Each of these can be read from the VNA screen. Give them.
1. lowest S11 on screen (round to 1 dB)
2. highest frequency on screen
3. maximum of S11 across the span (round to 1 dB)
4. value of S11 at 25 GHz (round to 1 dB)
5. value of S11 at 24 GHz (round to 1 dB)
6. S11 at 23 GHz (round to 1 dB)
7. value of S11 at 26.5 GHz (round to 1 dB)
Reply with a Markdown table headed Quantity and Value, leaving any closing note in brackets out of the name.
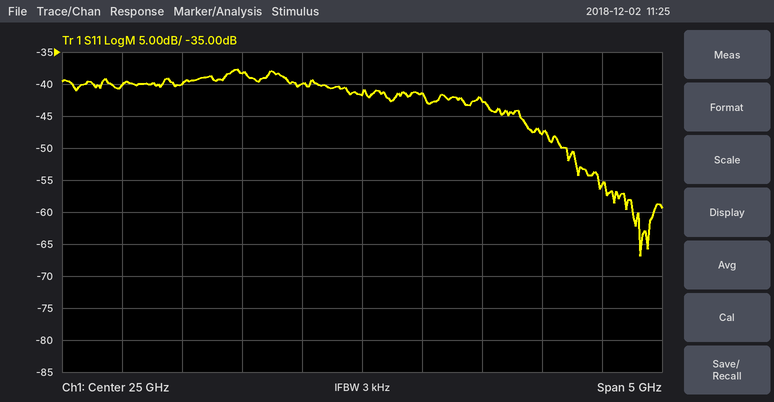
| Quantity | Value |
|---|---|
| lowest S11 on screen | -67 dB |
| highest frequency on screen | 27.5 GHz |
| maximum of S11 across the span | -38 dB |
| value of S11 at 25 GHz | -42 dB |
| value of S11 at 24 GHz | -38 dB |
| S11 at 23 GHz | -40 dB |
| value of S11 at 26.5 GHz | -48 dB |
